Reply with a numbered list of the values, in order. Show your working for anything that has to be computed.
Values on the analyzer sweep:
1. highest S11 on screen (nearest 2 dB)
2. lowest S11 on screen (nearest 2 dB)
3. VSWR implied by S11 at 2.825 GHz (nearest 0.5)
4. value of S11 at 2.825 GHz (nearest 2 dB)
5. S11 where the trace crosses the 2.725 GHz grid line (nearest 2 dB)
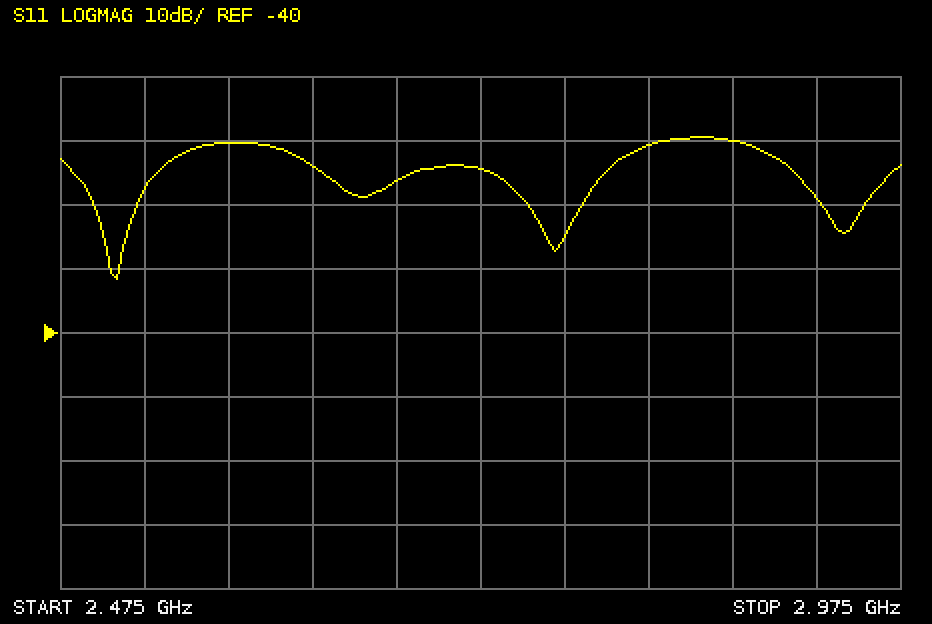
1. -10 dB
2. -32 dB
3. |Γ| = 10^(-10/20) = 0.3162; VSWR = (1 + 0.3162)/(1 − 0.3162) ≈ 1.92, so 2.0 to the nearest 0.5
4. -10 dB
5. -14 dB
